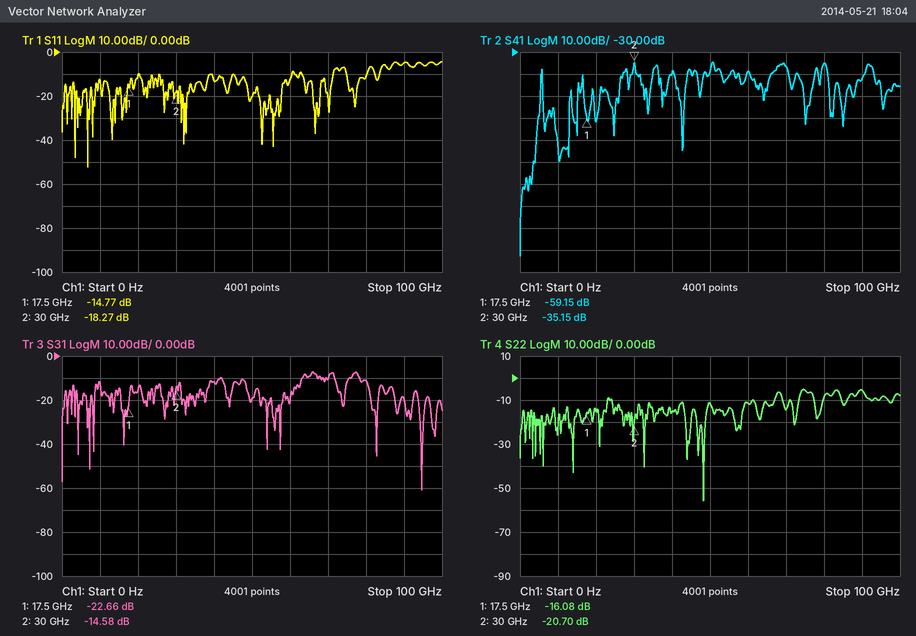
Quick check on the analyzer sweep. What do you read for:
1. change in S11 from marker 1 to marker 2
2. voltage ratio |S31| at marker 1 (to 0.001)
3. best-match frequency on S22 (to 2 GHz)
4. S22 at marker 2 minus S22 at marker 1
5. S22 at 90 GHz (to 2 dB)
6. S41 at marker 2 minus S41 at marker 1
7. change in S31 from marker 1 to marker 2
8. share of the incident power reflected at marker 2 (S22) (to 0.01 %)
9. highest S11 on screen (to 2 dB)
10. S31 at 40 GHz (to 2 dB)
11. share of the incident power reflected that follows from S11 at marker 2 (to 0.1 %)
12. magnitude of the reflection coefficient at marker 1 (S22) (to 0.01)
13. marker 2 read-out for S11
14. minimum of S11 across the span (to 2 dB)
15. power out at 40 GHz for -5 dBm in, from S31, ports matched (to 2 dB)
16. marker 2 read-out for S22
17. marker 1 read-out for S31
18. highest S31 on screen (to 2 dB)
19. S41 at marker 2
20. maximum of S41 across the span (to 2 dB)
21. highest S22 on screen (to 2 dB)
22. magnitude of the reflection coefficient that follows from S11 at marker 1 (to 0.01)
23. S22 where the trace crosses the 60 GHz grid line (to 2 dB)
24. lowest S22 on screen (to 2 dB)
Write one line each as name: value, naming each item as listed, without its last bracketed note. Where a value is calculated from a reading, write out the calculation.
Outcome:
change in S11 from marker 1 to marker 2: -18.27 − (-14.77) = -3.50 dB
voltage ratio |S31| at marker 1: 10^(-22.66/20) ≈ 0.074
best-match frequency on S22: 48 GHz
S22 at marker 2 minus S22 at marker 1: -20.7 − (-16.08) = -4.62 dB
S22 at 90 GHz: -6 dB
S41 at marker 2 minus S41 at marker 1: -35.15 − (-59.15) = 24.00 dB
change in S31 from marker 1 to marker 2: -14.58 − (-22.66) = 8.08 dB
share of the incident power reflected at marker 2 (S22): 10^(-20.7/10) ≈ 0.85 %
highest S11 on screen: -4 dB
S31 at 40 GHz: -12 dB
share of the incident power reflected that follows from S11 at marker 2: 10^(-18.27/10) ≈ 1.5 %
magnitude of the reflection coefficient at marker 1 (S22): 10^(-16.08/20) ≈ 0.16
marker 2 read-out for S11: -18.27 dB
minimum of S11 across the span: -52 dB
power out at 40 GHz for -5 dBm in, from S31, ports matched: -5 dBm + (-12 dB) = -16 dBm
marker 2 read-out for S22: -20.70 dB
marker 1 read-out for S31: -22.66 dB
highest S31 on screen: -8 dB
S41 at marker 2: -35.15 dB
maximum of S41 across the span: -34 dB
highest S22 on screen: -6 dB
magnitude of the reflection coefficient that follows from S11 at marker 1: 10^(-14.77/20) ≈ 0.18
S22 where the trace crosses the 60 GHz grid line: -12 dB
lowest S22 on screen: -56 dB
